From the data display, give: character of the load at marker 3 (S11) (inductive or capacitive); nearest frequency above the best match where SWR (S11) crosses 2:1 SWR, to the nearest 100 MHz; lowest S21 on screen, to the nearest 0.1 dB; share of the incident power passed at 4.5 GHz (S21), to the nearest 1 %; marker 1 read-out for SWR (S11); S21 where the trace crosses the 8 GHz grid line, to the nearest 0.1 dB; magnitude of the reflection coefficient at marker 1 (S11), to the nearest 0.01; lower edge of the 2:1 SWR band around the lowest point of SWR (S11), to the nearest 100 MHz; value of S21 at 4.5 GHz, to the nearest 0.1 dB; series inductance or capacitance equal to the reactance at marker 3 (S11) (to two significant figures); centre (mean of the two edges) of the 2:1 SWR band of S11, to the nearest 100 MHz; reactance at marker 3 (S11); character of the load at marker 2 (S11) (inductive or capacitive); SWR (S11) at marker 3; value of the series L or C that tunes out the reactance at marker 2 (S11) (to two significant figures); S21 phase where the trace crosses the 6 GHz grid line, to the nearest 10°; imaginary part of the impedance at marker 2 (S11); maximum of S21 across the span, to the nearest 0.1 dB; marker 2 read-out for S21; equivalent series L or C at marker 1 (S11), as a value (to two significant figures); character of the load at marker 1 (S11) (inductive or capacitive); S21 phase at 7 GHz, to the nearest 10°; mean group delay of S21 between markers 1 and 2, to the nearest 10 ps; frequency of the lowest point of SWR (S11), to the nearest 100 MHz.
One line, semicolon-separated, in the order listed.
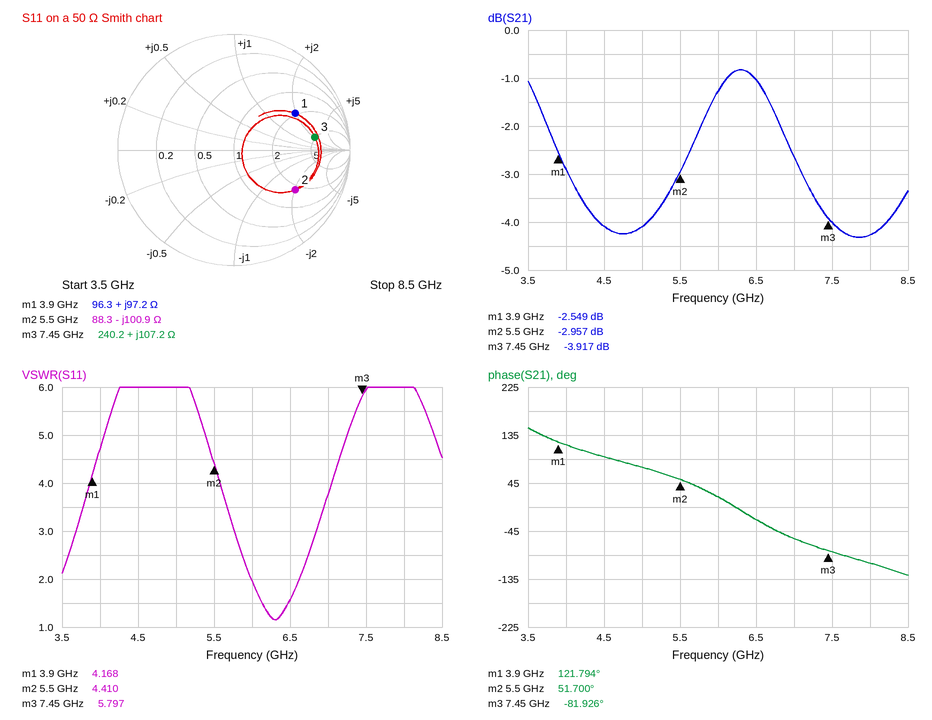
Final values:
inductive; 6.6 GHz; -4.3 dB; 39 %; 4.168; -4.3 dB; 0.61; 6.0 GHz; -4.1 dB; 2.3 nH; 6.3 GHz; +107.2 Ω; capacitive; 5.797; 2.9 nH; 20°; -100.9 Ω; -0.8 dB; -2.957 dB; 4.0 nH; inductive; -60°; 120 ps; 6.3 GHz
